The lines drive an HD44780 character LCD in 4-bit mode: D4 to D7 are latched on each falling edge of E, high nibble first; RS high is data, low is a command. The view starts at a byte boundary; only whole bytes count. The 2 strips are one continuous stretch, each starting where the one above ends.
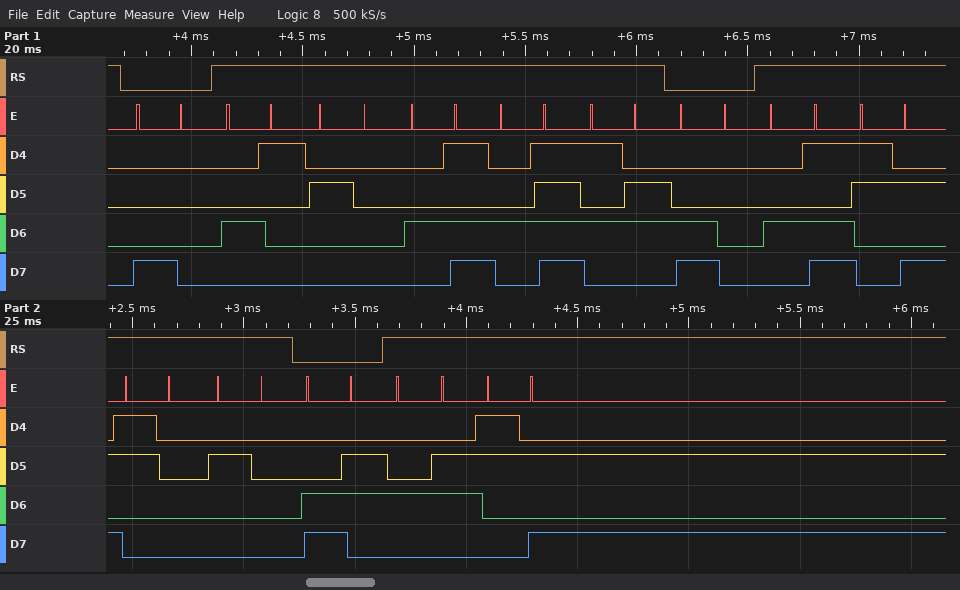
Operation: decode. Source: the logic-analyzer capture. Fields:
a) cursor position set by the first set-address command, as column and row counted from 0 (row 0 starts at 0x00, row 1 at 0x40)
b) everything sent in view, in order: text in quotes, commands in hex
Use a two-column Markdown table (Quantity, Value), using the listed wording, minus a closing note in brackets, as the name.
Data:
| Quantity | Value |
|---|---|
| cursor position set by the first set-address command, as column and row counted from 0 | column 0, row 0 |
| everything sent in view, in order: text in quotes, commands in hex | 0x80 "A MOV" 0xC0 "M:0 " 0xC6 "F:" |
